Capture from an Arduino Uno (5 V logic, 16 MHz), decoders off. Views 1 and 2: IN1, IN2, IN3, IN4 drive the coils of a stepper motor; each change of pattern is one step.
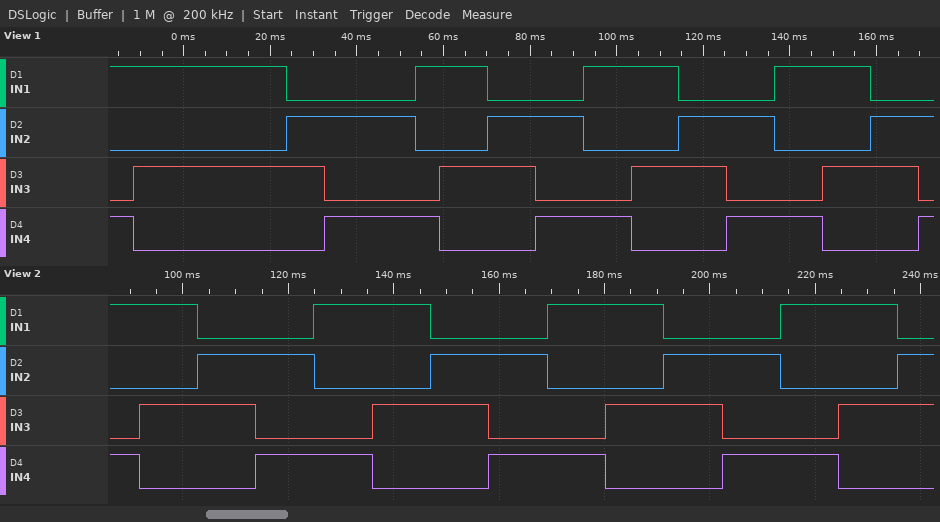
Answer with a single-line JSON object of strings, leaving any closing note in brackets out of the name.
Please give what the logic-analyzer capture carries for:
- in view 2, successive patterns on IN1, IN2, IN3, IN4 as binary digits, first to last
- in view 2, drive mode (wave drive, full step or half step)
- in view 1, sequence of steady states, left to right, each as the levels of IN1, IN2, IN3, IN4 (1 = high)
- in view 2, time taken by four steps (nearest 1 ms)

{"in view 2, successive patterns on IN1, IN2, IN3, IN4 as binary digits, first to last": "1001 1010 0110 0101 1001 1010 0110 0101 1001 1010 0110 0101 1001 1010 0110", "in view 2, drive mode": "full step", "in view 1, sequence of steady states, left to right, each as the levels of IN1, IN2, IN3, IN4": "1001 1010 0110 0101 1001 1010 0110 0101 1001 1010 0110 0101 1001 1010 0110 0101", "in view 2, time taken by four steps": "44 ms"}
